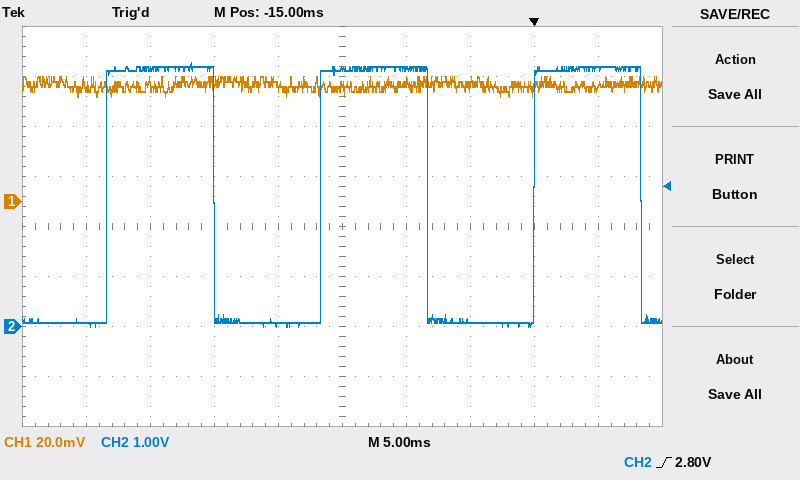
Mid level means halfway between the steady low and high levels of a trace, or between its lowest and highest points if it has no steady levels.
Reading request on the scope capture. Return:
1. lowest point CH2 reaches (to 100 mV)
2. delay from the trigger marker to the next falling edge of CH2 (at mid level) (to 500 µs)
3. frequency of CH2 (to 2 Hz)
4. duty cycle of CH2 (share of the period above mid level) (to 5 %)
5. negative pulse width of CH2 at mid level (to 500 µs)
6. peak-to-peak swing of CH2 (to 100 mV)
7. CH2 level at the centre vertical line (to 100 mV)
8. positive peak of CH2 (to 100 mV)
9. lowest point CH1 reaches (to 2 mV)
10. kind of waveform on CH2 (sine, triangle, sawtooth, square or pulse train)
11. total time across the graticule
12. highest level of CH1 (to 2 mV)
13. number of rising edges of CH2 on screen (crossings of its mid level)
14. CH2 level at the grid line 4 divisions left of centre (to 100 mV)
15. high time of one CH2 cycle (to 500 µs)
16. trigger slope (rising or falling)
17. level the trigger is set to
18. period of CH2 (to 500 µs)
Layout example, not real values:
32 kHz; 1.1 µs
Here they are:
0.0 V; 8.5 ms; 60 Hz; 50 %; 8.5 ms; 5.3 V; 5.2 V; 5.3 V; 42 mV; square; 50 ms; 50 mV; 3; 100 mV; 8.5 ms; rising; 2.80 V; 16.5 ms
